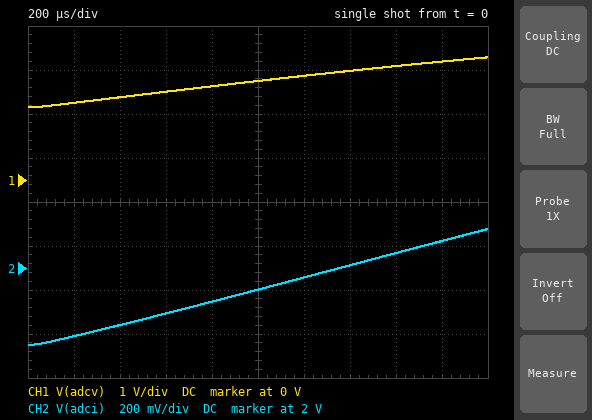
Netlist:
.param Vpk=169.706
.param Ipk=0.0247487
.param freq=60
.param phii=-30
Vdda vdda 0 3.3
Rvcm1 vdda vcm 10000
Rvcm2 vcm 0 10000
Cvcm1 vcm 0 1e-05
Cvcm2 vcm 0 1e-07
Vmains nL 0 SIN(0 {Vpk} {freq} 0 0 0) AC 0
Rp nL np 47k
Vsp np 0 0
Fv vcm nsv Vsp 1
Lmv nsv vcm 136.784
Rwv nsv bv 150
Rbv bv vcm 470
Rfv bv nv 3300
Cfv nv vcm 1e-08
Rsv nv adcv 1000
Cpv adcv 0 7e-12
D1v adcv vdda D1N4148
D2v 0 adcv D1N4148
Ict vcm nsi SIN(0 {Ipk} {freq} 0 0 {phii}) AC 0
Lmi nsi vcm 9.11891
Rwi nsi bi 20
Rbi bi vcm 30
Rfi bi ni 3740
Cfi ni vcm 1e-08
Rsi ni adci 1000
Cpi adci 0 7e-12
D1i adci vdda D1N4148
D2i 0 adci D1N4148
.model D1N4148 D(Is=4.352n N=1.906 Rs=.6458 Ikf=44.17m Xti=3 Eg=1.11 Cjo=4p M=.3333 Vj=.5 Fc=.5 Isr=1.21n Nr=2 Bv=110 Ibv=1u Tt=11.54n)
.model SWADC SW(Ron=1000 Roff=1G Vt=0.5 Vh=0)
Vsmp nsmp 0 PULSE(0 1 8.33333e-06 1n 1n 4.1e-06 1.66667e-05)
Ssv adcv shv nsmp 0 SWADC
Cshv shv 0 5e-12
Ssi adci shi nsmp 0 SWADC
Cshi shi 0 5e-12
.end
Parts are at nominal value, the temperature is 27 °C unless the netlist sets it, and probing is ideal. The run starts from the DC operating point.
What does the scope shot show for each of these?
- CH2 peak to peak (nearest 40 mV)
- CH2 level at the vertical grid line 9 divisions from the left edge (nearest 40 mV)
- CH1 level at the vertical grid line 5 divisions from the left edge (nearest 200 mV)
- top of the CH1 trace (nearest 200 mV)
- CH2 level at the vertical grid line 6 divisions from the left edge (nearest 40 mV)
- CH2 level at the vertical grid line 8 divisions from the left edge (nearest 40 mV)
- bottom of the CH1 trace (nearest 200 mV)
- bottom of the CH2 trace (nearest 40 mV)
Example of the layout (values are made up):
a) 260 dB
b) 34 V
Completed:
a) 520 mV
b) 2.12 V
c) 2.2 V
d) 2.8 V
e) 1.96 V
f) 2.08 V
g) 1.6 V
h) 1.64 V
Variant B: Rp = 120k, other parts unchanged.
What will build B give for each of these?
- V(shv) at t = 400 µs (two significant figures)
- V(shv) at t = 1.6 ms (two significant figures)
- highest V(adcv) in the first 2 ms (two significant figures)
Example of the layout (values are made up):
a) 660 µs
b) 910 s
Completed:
a) 1.7 V
b) 2.0 V
c) 2.1 V
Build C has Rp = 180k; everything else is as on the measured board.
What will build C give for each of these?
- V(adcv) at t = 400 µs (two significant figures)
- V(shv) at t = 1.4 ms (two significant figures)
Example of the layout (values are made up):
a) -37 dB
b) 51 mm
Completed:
a) 1.7 V
b) 1.9 V
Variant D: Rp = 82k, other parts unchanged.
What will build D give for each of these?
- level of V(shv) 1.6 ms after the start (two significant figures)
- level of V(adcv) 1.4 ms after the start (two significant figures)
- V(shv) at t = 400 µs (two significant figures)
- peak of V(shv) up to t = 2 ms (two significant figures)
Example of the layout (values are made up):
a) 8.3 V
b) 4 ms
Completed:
a) 2.2 V
b) 2.1 V
c) 1.8 V
d) 2.3 V
